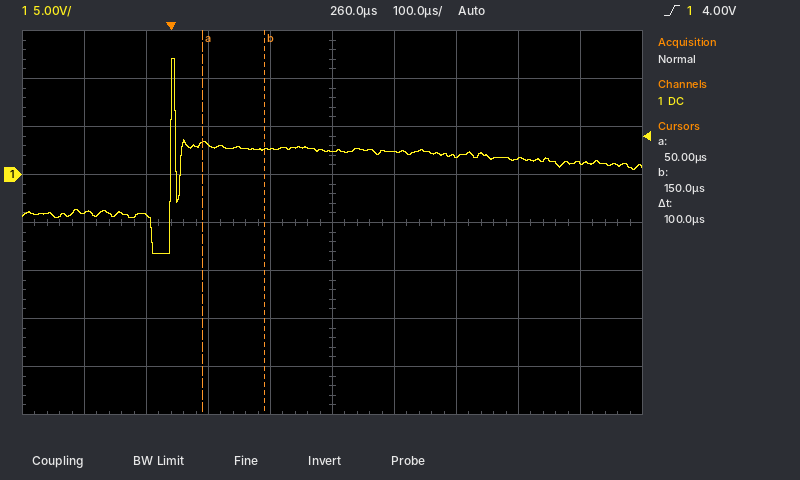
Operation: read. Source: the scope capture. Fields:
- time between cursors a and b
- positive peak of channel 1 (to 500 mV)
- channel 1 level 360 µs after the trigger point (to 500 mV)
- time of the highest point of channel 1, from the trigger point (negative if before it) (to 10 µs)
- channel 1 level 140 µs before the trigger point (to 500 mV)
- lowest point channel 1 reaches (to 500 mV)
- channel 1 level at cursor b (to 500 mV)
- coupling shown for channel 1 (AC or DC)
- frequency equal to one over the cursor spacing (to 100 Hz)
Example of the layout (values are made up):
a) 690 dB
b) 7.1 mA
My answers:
a) 100 µs
b) 12.0 V
c) 2.5 V
d) 0 µs
e) -4.0 V
f) -8.0 V
g) 2.5 V
h) DC
i) 10.0 kHz
